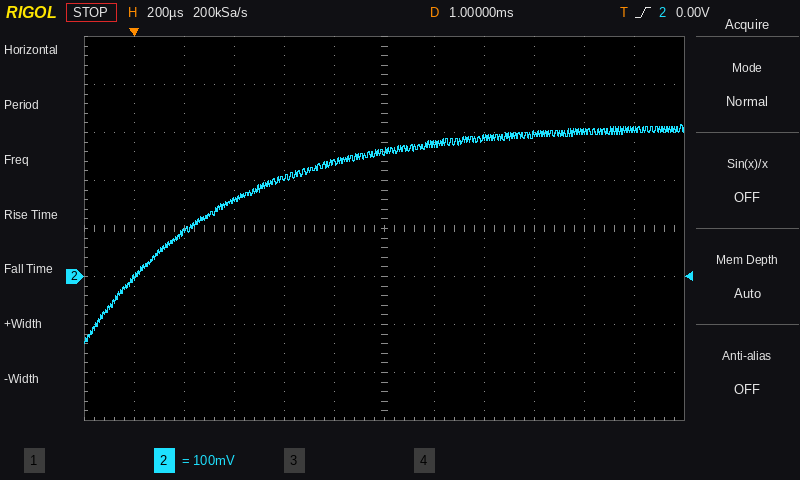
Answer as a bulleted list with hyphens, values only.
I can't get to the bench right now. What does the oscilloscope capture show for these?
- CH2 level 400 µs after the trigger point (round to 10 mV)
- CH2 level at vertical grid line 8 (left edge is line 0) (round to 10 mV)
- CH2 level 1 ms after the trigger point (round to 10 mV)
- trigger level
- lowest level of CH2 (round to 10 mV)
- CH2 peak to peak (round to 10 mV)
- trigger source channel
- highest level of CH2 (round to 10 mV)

- 160 mV
- 290 mV
- 260 mV
- 0.00 V
- -140 mV
- 460 mV
- CH2
- 320 mV
